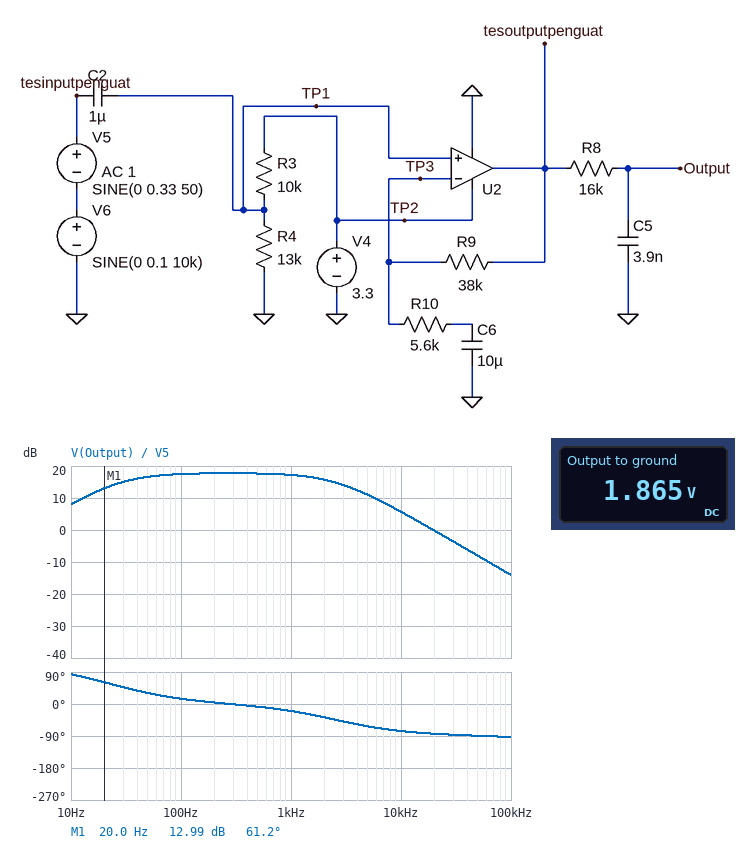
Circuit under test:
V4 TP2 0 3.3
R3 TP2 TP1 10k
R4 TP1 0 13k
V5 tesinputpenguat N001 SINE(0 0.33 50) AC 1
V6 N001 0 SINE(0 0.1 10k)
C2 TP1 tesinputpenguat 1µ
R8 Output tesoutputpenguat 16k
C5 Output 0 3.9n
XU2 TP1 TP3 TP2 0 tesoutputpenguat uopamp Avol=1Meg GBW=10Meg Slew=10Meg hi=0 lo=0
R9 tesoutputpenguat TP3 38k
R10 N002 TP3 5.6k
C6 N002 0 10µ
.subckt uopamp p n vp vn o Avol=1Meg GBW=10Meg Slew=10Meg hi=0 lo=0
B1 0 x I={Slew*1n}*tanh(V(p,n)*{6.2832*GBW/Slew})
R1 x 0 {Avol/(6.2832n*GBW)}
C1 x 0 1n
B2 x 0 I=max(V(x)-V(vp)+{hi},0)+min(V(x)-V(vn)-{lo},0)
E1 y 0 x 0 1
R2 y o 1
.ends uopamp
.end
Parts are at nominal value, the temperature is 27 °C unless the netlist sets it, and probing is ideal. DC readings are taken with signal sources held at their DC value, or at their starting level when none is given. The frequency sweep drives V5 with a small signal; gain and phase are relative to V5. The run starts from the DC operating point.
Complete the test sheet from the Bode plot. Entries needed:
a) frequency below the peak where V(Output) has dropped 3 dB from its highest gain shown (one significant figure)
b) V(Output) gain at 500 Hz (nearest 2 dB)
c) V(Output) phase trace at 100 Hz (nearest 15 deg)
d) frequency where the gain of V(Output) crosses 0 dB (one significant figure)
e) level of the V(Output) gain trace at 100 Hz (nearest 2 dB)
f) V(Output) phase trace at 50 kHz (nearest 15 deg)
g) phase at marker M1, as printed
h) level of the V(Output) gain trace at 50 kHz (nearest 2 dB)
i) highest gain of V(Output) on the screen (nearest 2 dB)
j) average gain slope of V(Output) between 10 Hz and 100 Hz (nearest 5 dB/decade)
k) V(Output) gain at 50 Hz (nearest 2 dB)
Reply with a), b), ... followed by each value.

a) 30 Hz
b) 18 dB
c) 15 deg
d) 20 kHz
e) 18 dB
f) -90 deg
g) 61.2 deg
h) -8 dB
i) 18 dB
j) 10 dB/decade
k) 16 dB
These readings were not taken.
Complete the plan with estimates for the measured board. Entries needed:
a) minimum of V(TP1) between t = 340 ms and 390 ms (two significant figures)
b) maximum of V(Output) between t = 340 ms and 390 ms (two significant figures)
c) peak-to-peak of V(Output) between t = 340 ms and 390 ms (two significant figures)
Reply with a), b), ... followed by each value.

a) 1.5 V
b) 3.3 V
c) 3.2 V
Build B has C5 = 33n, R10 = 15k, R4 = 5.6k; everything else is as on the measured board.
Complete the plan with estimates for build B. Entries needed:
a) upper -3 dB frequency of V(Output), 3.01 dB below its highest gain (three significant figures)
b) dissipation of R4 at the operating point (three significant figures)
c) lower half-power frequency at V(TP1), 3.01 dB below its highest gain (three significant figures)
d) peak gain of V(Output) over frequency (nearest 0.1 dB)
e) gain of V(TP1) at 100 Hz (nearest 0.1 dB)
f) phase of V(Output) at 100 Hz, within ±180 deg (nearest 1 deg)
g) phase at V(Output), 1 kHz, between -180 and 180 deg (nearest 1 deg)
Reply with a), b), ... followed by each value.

a) 381 Hz
b) 251 µW
c) 44.3 Hz
d) 9.8 dB
e) -0.8 dB
f) 6 deg
g) -71 deg
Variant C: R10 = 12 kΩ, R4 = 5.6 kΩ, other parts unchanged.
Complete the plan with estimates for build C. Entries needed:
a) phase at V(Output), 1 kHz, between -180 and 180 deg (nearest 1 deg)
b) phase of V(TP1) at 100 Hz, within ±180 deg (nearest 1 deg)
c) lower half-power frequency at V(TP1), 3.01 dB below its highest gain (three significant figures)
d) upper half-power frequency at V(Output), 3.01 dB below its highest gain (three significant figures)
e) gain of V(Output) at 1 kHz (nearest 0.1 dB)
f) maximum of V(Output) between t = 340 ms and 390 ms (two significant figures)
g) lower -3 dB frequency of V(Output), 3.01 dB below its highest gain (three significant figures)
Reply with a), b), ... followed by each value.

a) -19 deg
b) 24 deg
c) 44.3 Hz
d) 2.64 kHz
e) 11.8 dB
f) 2.3 V
g) 42.9 Hz
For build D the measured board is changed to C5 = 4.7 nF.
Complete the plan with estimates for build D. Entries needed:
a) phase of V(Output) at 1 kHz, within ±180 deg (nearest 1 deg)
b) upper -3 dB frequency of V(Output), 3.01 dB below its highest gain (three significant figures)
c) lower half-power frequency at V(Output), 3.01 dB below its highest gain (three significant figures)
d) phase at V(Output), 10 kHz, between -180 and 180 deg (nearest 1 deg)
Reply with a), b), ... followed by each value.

a) -24 deg
b) 2.17 kHz
c) 27.7 Hz
d) -78 deg
